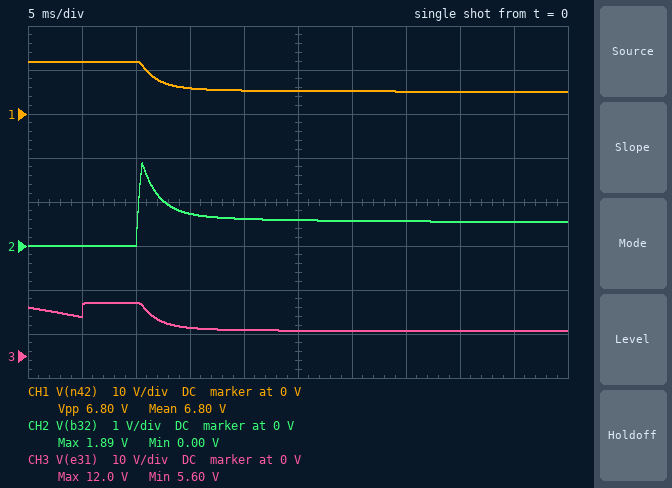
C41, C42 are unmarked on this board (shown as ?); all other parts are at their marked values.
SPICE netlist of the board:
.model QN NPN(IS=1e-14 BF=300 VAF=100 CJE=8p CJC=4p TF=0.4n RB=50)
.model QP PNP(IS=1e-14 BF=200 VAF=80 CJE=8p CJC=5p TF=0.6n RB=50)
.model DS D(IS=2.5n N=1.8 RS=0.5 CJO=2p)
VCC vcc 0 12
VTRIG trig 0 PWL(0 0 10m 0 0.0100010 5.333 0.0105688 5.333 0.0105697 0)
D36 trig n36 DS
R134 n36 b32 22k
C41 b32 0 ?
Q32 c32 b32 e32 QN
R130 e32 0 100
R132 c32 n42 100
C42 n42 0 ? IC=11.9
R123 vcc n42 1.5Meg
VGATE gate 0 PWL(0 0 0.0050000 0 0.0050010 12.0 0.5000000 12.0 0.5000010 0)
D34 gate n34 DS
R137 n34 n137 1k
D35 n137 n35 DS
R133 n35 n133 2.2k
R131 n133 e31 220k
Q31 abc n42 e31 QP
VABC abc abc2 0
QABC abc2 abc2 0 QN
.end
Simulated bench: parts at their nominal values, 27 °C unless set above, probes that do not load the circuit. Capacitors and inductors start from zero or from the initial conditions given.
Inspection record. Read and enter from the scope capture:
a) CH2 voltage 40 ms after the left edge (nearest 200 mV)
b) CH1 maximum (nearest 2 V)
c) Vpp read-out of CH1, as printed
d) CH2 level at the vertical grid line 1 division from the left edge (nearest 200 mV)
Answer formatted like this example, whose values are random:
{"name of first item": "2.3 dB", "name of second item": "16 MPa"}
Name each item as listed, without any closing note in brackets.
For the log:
{"CH2 voltage 40 ms after the left edge": "600 mV", "CH1 maximum": "12 V", "Vpp read-out of CH1, as printed": "6.80 V", "CH2 level at the vertical grid line 1 division from the left edge": "0 V"}
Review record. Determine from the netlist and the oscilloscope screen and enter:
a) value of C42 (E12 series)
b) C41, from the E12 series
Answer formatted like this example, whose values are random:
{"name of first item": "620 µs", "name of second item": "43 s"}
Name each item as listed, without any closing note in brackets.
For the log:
{"value of C42": "3.3 µF", "C41, from the E12 series": "47 nF"}
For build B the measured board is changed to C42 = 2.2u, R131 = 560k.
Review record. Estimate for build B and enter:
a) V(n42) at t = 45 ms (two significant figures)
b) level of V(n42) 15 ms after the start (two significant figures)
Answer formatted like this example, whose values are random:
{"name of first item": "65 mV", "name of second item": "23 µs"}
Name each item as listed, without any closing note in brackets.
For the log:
{"V(n42) at t = 45 ms": "1.8 V", "level of V(n42) 15 ms after the start": "2.9 V"}
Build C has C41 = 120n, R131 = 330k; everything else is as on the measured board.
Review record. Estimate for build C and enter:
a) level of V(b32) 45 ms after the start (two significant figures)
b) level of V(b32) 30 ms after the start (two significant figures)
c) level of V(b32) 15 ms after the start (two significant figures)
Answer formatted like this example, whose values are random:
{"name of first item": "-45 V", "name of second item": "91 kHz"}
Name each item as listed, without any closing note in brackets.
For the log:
{"level of V(b32) 45 ms after the start": "580 mV", "level of V(b32) 30 ms after the start": "610 mV", "level of V(b32) 15 ms after the start": "750 mV"}
